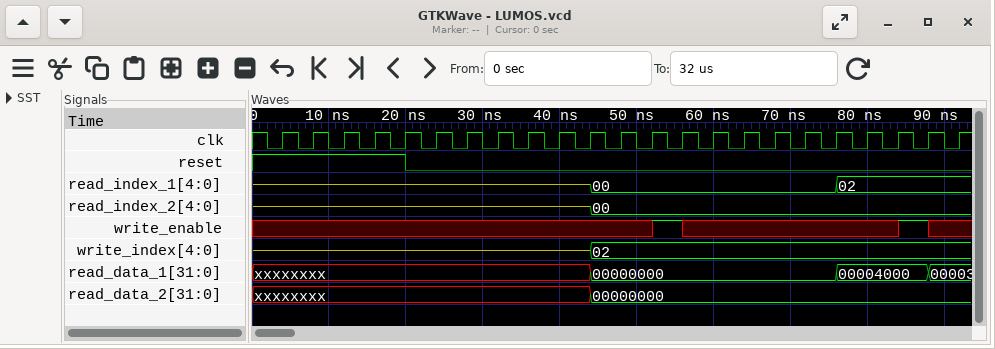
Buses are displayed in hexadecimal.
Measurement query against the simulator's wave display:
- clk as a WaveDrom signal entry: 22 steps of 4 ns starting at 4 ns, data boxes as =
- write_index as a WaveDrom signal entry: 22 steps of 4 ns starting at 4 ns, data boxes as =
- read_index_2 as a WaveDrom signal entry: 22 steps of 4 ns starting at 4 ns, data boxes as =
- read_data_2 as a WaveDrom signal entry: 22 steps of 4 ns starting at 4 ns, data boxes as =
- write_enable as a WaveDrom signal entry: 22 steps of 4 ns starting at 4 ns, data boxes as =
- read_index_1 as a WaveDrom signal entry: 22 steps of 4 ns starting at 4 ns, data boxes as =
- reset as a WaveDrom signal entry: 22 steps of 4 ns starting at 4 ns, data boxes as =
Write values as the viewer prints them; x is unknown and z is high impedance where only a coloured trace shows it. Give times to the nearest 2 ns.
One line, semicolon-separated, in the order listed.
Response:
{name: 'clk', wave: 'p.....................'}; {name: 'write_index', wave: 'z.........=...........', data: '02'}; {name: 'read_index_2', wave: 'z.........=...........', data: '00'}; {name: 'read_data_2', wave: 'x.........=...........', data: '00000000'}; {name: 'write_enable', wave: 'x...........1x......1x'}; {name: 'read_index_1', wave: 'z.........=.......=...', data: '00 02'}; {name: 'reset', wave: '1...0.................'}
